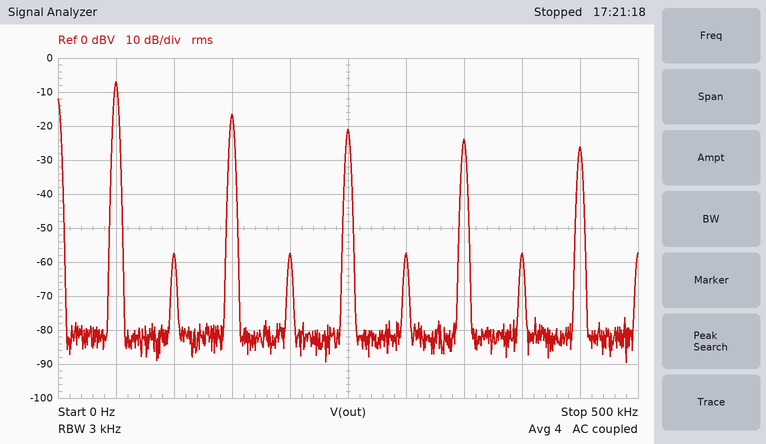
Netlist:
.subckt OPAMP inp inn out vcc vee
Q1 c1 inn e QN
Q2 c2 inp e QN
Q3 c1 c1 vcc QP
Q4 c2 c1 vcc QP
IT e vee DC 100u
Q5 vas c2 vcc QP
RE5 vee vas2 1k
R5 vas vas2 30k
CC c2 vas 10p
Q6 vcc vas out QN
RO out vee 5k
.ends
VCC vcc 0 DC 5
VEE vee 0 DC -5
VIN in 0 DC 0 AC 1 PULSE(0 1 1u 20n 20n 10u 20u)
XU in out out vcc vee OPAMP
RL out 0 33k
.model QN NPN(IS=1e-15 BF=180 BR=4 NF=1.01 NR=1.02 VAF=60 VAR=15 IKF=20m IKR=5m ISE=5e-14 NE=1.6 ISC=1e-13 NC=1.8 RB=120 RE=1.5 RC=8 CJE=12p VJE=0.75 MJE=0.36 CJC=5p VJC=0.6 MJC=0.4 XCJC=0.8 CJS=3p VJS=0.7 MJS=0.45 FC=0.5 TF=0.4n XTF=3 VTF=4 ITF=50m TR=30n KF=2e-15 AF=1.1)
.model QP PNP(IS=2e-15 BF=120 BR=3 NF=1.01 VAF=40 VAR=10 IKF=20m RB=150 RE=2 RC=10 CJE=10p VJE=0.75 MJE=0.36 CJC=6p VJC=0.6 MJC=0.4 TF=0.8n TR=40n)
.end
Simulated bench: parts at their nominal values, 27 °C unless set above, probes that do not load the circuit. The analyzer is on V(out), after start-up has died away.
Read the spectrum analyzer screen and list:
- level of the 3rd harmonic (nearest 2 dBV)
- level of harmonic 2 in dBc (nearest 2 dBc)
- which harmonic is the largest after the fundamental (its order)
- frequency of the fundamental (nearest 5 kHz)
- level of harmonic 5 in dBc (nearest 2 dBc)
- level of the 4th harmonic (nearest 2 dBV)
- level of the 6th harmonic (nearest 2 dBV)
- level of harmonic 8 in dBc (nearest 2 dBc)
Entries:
-16 dBV
-50 dBc
3
50 kHz
-14 dBc
-58 dBV
-58 dBV
-50 dBc
